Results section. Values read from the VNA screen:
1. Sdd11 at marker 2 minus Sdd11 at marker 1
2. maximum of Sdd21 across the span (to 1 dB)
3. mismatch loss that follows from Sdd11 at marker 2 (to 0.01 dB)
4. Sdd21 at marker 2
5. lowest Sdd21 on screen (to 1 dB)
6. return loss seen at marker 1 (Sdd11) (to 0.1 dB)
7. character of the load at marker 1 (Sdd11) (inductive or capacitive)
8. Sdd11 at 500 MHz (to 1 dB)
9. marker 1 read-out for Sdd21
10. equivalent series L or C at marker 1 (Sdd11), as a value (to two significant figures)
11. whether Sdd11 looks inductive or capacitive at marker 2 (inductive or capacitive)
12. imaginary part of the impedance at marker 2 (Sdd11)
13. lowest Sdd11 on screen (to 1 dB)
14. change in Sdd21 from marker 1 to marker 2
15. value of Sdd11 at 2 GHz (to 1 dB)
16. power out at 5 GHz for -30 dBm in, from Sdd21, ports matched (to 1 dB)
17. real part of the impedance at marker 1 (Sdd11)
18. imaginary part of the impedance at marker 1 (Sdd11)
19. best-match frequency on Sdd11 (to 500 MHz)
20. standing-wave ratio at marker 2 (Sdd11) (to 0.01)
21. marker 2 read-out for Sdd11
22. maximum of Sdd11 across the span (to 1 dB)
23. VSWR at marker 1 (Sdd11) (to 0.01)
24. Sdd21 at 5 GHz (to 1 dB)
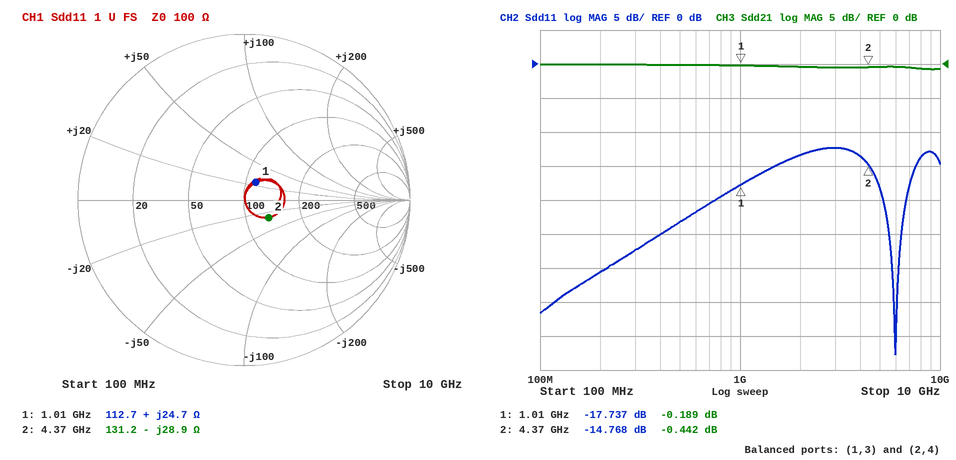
2.969 dB
0 dB
0.15 dB
-0.442 dB
-1 dB
17.7 dB
inductive
-23 dB
-0.189 dB
3.9 nH
capacitive
-28.9 Ω
-43 dB
-0.253 dB
-13 dB
-30 dBm
112.7 Ω
+24.7 Ω
6.0 GHz
1.45
-14.768 dB
-12 dB
1.30
0 dB
